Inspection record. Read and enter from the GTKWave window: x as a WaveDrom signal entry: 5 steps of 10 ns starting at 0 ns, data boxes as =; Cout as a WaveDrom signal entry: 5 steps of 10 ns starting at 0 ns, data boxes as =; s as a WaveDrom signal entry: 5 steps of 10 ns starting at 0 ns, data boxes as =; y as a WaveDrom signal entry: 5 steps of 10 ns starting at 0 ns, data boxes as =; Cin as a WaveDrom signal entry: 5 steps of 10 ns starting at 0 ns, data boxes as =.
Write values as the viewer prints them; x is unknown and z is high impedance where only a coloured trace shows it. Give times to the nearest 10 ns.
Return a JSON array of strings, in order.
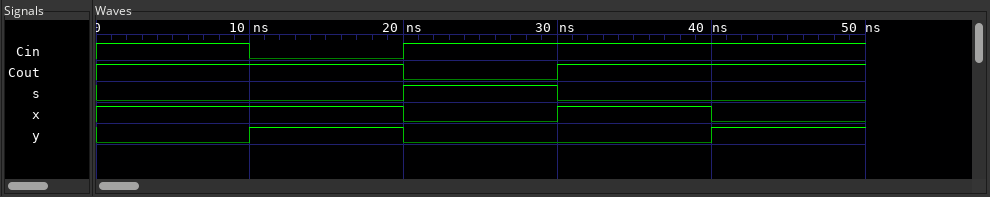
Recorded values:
["{name: 'x', wave: '1.010'}", "{name: 'Cout', wave: '1.01.'}", "{name: 's', wave: '0.10.'}", "{name: 'y', wave: '010.1'}", "{name: 'Cin', wave: '101..'}"]
